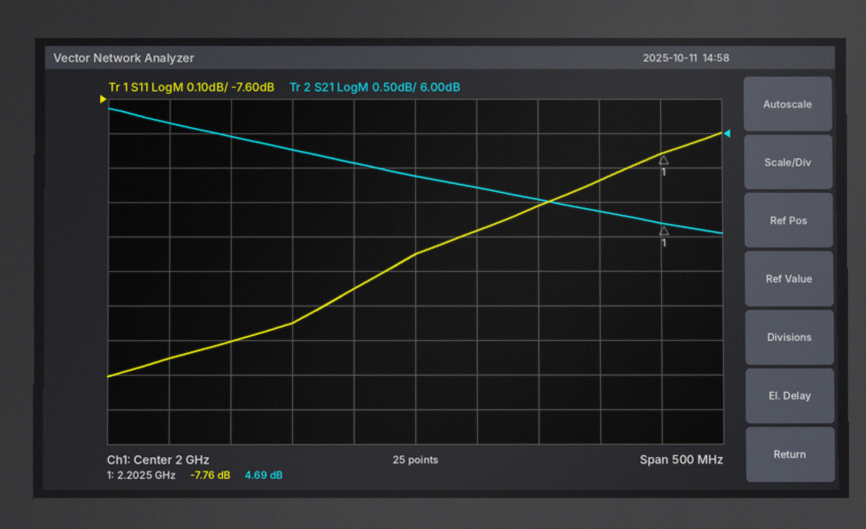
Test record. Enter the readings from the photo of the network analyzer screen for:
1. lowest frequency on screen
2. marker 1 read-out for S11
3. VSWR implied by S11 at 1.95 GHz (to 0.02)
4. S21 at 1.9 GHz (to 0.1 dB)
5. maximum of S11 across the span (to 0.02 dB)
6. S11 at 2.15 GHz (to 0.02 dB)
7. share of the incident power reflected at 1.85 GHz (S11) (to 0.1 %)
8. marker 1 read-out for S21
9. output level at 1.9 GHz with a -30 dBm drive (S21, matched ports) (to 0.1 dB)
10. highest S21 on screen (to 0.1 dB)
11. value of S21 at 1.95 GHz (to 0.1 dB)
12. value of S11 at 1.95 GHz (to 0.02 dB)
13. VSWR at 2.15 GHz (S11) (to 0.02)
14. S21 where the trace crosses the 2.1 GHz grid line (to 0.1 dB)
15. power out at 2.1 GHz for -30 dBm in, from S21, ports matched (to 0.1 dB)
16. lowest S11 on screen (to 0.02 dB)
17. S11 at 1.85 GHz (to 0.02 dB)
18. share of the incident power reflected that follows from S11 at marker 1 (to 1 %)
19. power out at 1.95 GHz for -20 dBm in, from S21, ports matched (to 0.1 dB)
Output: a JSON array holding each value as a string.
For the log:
["1.75 GHz", "-7.76 dB", "2.28", "5.8 dB", "-7.70 dB", "-7.84 dB", "14.8 %", "4.69 dB", "-24.2 dBm", "6.4 dB", "5.6 dB", "-8.16 dB", "2.36", "5.0 dB", "-25.0 dBm", "-8.40 dB", "-8.30 dB", "17 %", "-14.4 dBm"]
